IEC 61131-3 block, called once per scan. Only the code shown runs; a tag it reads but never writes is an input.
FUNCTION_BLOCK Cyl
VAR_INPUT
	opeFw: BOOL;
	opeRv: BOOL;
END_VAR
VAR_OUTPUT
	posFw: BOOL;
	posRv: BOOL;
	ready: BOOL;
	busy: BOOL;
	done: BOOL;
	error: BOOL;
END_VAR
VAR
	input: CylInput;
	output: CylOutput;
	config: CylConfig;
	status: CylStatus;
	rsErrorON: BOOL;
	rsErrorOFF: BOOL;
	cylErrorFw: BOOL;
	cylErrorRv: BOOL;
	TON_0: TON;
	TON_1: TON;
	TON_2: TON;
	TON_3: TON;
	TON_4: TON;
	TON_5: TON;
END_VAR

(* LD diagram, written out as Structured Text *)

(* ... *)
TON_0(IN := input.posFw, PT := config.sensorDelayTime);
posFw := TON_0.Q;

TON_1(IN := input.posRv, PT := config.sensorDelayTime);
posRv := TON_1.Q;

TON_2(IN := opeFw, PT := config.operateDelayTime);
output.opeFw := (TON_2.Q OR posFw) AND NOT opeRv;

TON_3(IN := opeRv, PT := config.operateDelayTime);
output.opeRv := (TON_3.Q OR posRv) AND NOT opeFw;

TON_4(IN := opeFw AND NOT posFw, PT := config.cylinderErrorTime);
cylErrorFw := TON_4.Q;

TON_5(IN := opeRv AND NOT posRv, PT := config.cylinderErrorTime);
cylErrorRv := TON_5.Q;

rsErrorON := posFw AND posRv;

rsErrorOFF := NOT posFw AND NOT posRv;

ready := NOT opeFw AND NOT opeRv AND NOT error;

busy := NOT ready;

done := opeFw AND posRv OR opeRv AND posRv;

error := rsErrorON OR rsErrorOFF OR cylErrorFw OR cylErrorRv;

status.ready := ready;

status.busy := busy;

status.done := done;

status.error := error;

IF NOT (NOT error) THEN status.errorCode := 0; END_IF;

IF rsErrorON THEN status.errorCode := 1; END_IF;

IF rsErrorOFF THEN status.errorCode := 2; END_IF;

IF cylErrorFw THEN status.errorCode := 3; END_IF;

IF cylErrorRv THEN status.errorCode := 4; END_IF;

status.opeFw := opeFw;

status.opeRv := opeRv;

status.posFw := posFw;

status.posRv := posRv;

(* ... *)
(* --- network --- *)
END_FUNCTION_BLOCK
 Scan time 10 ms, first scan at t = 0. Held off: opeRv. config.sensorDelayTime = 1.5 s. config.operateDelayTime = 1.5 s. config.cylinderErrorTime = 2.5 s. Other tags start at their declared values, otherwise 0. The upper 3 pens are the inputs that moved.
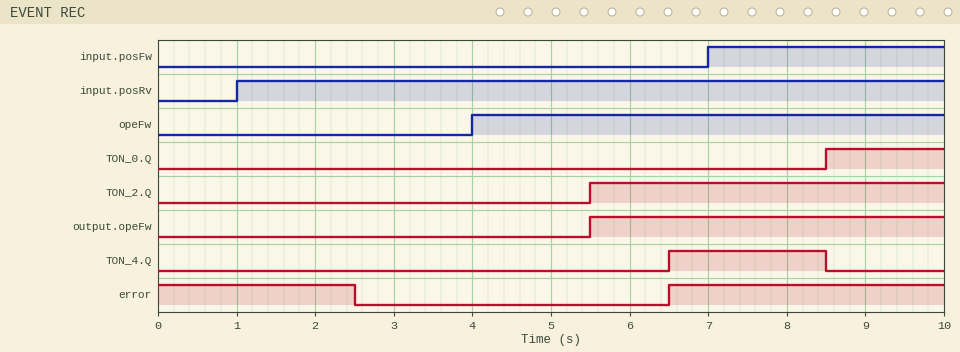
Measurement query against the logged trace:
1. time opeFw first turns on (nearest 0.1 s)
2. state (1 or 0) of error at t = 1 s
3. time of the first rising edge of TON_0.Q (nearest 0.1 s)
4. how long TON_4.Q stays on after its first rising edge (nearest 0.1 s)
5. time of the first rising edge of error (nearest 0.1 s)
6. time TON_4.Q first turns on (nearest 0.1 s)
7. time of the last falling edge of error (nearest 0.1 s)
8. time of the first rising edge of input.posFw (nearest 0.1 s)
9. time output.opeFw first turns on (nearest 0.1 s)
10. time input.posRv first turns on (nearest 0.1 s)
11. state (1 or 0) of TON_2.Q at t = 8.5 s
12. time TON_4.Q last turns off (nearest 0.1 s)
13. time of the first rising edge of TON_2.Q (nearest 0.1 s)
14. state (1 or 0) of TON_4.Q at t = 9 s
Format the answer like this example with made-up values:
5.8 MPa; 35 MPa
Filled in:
4.0 s; 1; 8.5 s; 2.0 s; 6.5 s; 6.5 s; 2.5 s; 7.0 s; 5.5 s; 1.0 s; 1; 8.5 s; 5.5 s; 0
